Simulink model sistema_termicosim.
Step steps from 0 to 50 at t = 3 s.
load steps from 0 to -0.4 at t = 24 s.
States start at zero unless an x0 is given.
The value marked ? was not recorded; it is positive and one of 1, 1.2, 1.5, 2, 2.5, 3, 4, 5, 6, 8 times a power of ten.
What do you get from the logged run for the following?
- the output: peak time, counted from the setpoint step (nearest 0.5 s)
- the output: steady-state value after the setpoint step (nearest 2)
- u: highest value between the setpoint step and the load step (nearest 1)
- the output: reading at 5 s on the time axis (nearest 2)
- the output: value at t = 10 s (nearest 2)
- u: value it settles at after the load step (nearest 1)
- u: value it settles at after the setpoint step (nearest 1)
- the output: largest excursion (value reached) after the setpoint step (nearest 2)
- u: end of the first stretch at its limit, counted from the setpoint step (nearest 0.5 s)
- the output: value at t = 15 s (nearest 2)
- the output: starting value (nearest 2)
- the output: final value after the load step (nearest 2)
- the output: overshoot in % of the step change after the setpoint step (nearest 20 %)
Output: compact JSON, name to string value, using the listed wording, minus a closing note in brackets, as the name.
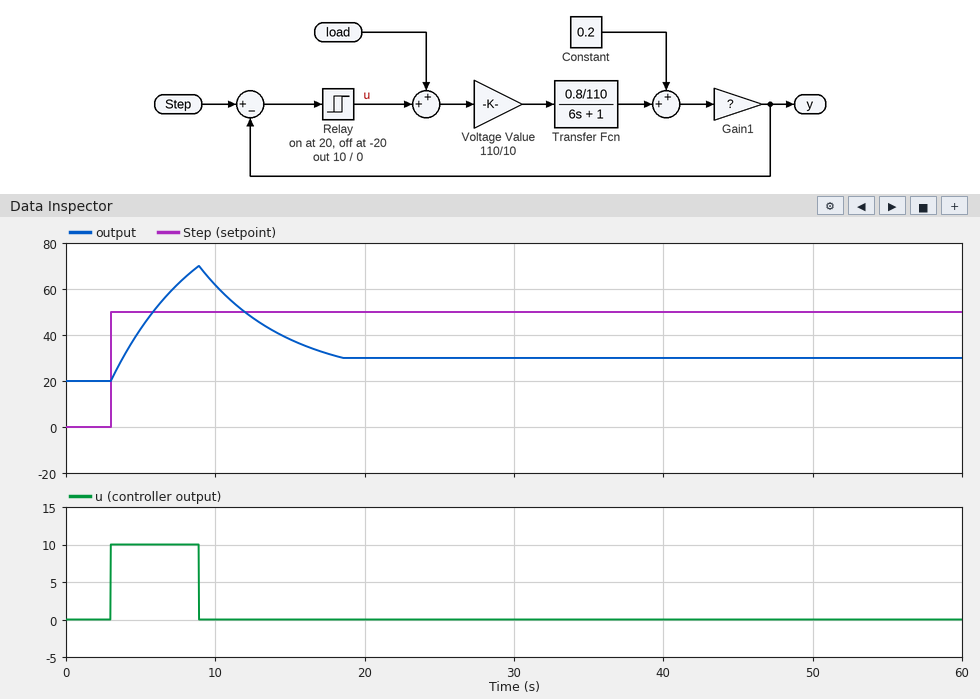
{"the output: peak time, counted from the setpoint step": "6.0 s", "the output: steady-state value after the setpoint step": "30", "u: highest value between the setpoint step and the load step": "10", "the output: reading at 5 s on the time axis": "42", "the output: value at t = 10 s": "62", "u: value it settles at after the load step": "0", "u: value it settles at after the setpoint step": "0", "the output: largest excursion (value reached) after the setpoint step": "70", "u: end of the first stretch at its limit, counted from the setpoint step": "6.0 s", "the output: value at t = 15 s": "38", "the output: starting value": "20", "the output: final value after the load step": "30", "the output: overshoot in % of the step change after the setpoint step": "400 %"}
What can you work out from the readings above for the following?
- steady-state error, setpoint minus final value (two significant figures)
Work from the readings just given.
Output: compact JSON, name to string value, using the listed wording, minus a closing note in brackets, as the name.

{"steady-state error, setpoint minus final value": "20"}
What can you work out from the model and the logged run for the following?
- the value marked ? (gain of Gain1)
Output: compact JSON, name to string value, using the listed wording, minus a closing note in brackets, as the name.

{"the value marked ?": "100"}
